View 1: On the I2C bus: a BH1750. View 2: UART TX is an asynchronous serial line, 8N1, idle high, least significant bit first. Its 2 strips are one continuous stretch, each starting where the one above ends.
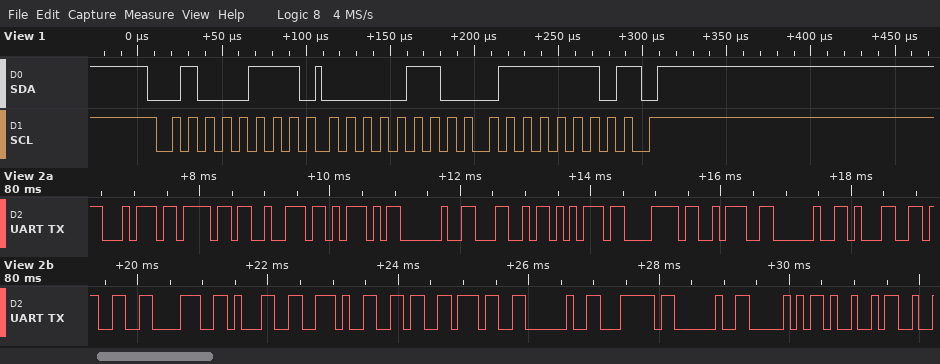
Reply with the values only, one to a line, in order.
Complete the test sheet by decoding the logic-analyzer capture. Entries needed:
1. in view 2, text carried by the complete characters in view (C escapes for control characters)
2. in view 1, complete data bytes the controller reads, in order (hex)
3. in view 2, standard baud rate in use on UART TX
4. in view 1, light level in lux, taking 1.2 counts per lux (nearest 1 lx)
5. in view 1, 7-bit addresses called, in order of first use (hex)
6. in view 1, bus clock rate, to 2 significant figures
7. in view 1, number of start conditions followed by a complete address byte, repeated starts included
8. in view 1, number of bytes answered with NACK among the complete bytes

"tor] Lux: 1381.67 | PI"
06 7E
9600 baud
1385 lx
0x23
100 kHz
1
1
